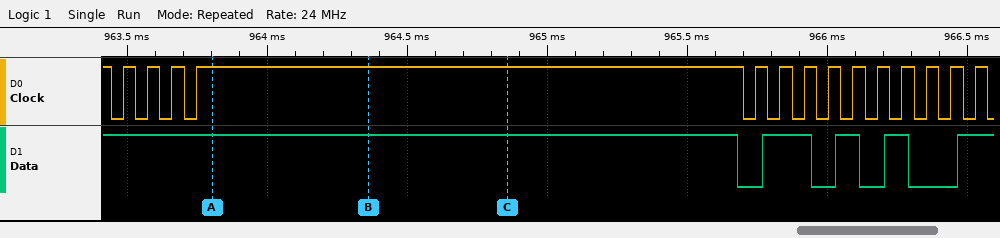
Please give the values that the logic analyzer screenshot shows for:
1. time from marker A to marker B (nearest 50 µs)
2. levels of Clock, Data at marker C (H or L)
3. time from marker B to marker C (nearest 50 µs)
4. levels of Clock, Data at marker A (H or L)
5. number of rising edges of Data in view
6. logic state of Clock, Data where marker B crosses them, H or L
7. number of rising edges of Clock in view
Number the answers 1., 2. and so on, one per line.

1. 550 µs
2. Clock=H, Data=H
3. 500 µs
4. Clock=H, Data=H
5. 4
6. Clock=H, Data=H
7. 14
